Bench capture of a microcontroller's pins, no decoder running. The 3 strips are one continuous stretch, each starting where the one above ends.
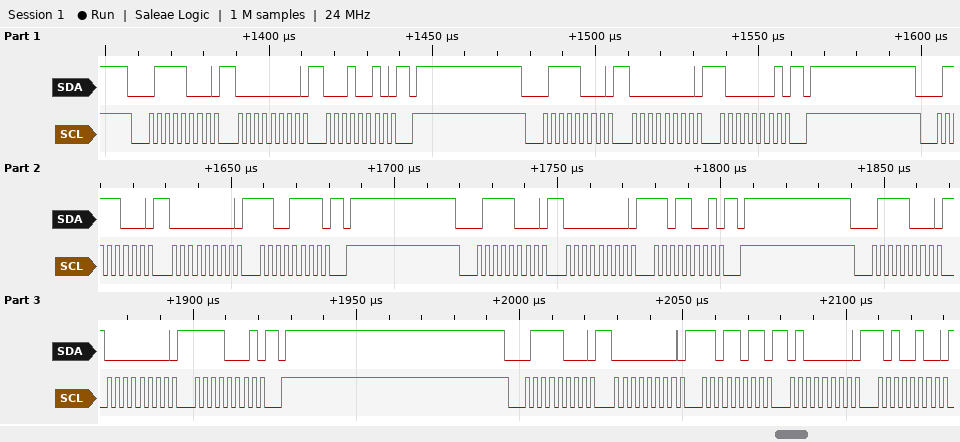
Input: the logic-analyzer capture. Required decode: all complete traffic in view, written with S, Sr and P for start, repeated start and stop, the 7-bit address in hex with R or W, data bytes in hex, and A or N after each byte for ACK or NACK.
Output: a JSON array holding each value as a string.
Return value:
["S 3CW A 00 A 12 A P S 3CW A 00 A 81 A P S 3CW A 00 A CF A P S 3CW A 00 A D9 A P S 3CW A 00 A F1 A P S 3CW A 00 A DB A 40 A A4 A"]
